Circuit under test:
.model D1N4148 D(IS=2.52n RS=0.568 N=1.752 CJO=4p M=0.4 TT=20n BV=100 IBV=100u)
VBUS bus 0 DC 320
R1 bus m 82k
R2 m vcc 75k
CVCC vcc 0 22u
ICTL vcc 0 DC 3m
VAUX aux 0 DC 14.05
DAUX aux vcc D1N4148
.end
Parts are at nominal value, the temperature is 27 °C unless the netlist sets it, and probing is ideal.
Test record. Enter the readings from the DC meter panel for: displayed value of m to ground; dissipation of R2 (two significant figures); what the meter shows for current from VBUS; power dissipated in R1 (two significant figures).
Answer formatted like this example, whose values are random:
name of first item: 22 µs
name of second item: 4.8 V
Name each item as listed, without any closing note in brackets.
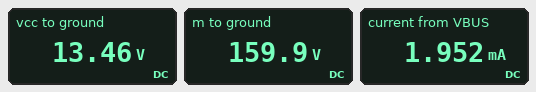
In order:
displayed value of m to ground: 159.9 V
dissipation of R2: 290 mW
what the meter shows for current from VBUS: 1.952 mA
power dissipated in R1: 310 mW
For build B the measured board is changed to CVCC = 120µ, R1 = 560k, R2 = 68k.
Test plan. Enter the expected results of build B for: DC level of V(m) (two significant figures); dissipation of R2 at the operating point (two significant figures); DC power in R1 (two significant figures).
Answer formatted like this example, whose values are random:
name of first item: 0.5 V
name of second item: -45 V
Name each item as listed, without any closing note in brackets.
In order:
DC level of V(m): 47 V
dissipation of R2 at the operating point: 16 mW
DC power in R1: 130 mW
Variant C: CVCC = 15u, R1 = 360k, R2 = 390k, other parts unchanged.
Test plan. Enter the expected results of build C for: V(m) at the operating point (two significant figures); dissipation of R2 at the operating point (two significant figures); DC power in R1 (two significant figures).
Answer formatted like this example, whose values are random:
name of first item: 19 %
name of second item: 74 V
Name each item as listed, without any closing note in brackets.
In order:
V(m) at the operating point: 170 V
dissipation of R2 at the operating point: 65 mW
DC power in R1: 60 mW
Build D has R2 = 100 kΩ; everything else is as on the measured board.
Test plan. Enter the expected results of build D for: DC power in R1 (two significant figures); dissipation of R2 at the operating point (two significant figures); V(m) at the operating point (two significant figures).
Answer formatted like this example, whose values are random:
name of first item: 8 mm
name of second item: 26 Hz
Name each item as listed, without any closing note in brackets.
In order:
DC power in R1: 230 mW
dissipation of R2 at the operating point: 280 mW
V(m) at the operating point: 180 V
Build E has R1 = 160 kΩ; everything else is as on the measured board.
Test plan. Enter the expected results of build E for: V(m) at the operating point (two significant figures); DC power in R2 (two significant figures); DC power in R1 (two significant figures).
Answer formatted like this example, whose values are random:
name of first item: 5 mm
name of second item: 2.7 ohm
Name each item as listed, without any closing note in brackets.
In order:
V(m) at the operating point: 110 V
DC power in R2: 130 mW
DC power in R1: 270 mW
